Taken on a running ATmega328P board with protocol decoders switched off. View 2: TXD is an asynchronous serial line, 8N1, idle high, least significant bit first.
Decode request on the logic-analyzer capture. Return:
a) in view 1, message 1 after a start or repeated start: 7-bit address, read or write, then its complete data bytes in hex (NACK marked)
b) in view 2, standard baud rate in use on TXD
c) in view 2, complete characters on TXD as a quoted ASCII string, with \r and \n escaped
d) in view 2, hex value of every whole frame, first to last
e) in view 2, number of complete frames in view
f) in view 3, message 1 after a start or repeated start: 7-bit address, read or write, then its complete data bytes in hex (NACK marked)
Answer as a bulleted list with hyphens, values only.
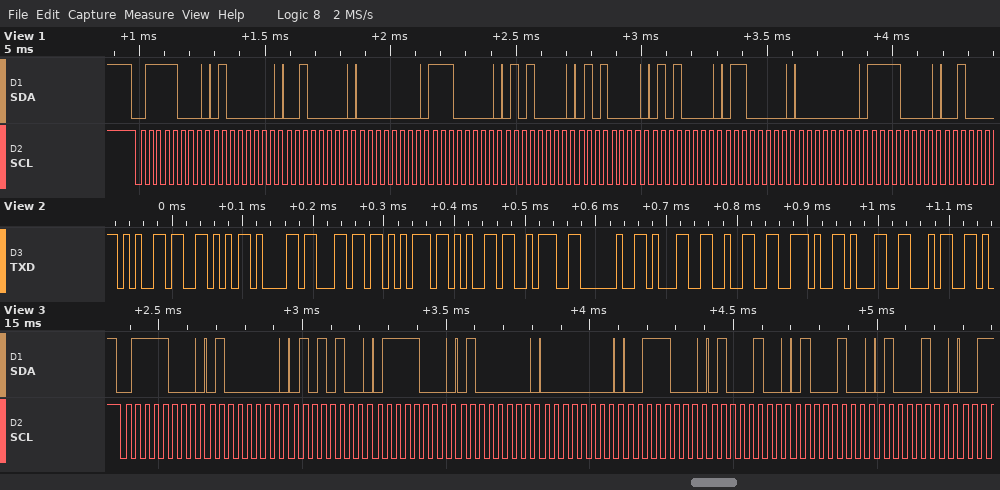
- 0x3C write: 40 20 00 E0 50 50 50 60 00 F0
- 115200 baud
- "eValue: 12.14"
- 65 56 61 6C 75 65 3A 20 31 32 2E 31 34
- 13
- 0x3C write: 40 54 78 40 00 38 44 44 44
